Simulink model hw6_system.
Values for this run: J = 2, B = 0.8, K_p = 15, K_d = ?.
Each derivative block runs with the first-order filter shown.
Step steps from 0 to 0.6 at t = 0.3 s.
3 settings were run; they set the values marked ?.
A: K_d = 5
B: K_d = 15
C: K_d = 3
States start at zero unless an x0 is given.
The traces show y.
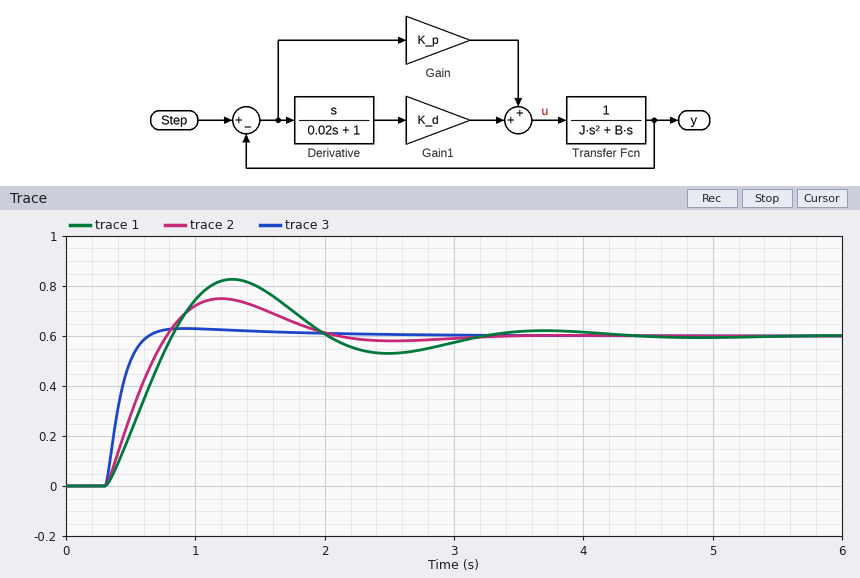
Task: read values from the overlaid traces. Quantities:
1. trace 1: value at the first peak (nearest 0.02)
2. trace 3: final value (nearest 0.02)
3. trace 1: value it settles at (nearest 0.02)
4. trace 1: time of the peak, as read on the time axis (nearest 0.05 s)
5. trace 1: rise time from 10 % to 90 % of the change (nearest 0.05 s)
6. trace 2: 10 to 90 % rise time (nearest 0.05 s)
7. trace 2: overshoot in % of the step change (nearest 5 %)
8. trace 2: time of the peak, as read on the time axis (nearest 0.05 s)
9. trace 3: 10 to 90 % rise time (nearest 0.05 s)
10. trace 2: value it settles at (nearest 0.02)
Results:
0.82
0.60
0.60
1.30 s
0.40 s
0.35 s
25 %
1.20 s
0.20 s
0.60
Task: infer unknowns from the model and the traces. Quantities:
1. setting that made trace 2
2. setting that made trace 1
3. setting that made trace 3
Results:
A
C
B
